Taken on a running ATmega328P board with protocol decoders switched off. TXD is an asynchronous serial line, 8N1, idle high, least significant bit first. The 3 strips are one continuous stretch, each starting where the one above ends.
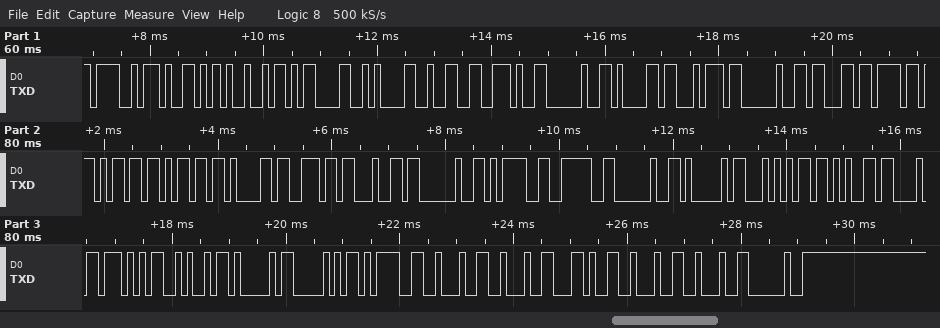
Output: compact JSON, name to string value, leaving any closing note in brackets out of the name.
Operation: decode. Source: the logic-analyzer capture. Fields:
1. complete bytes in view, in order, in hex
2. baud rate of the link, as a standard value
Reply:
{"complete bytes in view, in order, in hex": "4F 59 49 0D 0A 32 2E 20 61 74 20 63 6F 6D 6D 61 6E 64 20 3D 3E 20 41 54 2B 43 57 4A 41 50 3D 22 22 2C 22 22 20", "baud rate of the link, as a standard value": "9600 baud"}
